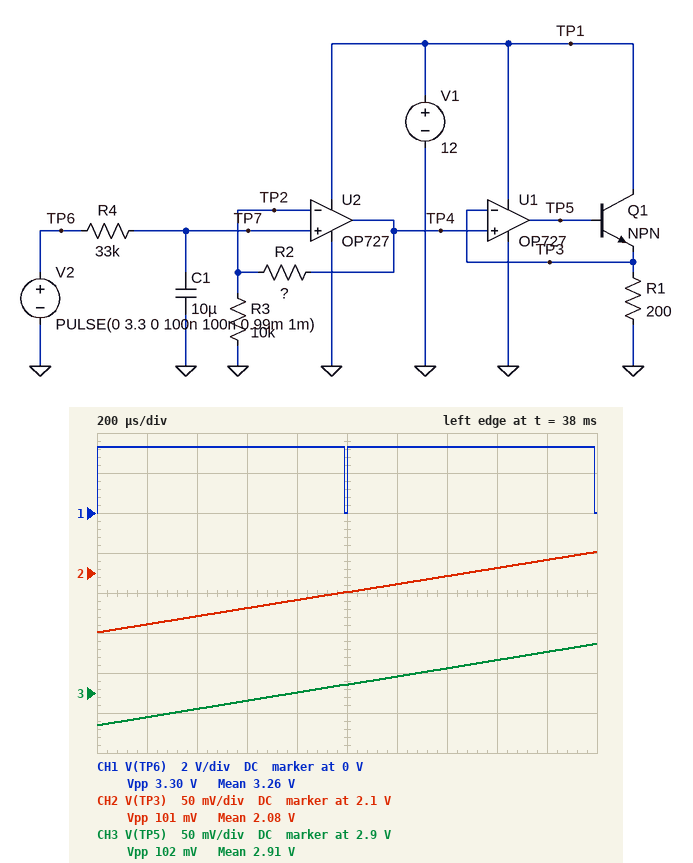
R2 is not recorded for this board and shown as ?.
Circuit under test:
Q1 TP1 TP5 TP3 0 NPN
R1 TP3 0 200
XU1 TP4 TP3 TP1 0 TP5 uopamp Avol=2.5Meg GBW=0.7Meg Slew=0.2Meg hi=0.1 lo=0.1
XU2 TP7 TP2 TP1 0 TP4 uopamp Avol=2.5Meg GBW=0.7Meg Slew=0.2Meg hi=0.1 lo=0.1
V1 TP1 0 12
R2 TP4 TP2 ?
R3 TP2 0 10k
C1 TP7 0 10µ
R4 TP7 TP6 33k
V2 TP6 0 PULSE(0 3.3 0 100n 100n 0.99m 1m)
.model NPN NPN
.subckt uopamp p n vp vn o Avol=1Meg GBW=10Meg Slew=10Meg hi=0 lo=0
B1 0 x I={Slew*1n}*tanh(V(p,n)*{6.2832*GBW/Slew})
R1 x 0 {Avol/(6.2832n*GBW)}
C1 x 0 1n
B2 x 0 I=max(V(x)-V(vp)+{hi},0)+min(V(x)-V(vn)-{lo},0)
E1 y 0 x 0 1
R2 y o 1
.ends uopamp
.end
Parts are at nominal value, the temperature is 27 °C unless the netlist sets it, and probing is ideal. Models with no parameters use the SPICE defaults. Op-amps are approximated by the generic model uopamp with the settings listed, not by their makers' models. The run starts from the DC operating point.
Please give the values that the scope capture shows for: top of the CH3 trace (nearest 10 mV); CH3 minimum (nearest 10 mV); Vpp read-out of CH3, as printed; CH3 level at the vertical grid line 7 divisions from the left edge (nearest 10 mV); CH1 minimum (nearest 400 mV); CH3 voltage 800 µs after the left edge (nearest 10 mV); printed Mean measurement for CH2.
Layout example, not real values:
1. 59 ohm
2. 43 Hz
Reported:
1. 2.96 V
2. 2.86 V
3. 102 mV
4. 2.93 V
5. 0 V
6. 2.90 V
7. 2.08 V
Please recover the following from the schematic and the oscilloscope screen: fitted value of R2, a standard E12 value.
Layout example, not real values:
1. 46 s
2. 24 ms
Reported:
1. 47 kΩ
